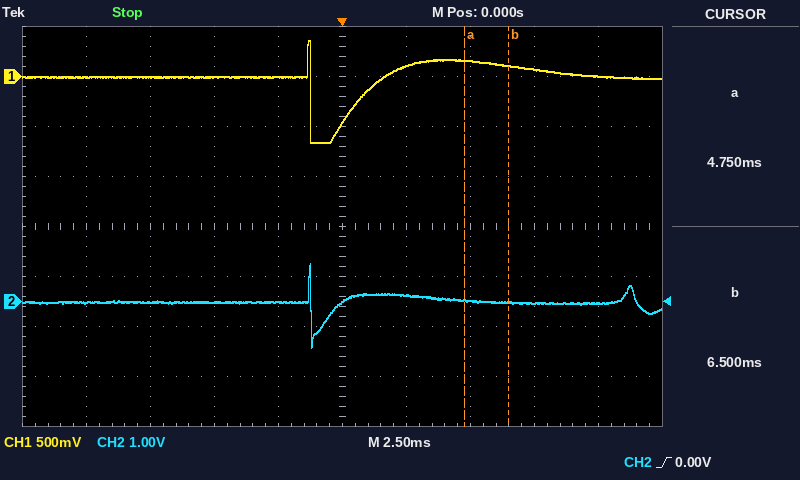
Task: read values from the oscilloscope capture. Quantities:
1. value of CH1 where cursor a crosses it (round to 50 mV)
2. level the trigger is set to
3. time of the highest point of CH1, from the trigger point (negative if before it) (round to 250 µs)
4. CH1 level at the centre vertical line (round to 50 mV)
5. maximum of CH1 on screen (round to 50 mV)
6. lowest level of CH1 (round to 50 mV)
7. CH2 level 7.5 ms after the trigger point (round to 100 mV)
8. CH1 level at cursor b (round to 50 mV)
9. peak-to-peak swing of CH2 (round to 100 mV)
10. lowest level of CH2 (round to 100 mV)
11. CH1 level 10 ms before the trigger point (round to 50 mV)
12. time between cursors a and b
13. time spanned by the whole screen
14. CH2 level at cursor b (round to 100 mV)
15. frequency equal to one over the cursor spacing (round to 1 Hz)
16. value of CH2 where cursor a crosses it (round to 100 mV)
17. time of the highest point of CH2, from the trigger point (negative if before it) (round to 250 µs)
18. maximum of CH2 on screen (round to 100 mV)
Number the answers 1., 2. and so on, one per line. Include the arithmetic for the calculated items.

1. 150 mV
2. 0.00 V
3. -1.25 ms
4. -450 mV
5. 350 mV
6. -650 mV
7. 0.0 V
8. 100 mV
9. 800 mV − (-900 mV) = 1.7 V
10. -900 mV
11. 0 mV
12. 6.5 ms − (4.75 ms) = 1.75 ms
13. 25 ms
14. 0.0 V
15. 1 / 1.75 ms ≈ 571 Hz
16. 0.0 V
17. -1.25 ms
18. 800 mV
